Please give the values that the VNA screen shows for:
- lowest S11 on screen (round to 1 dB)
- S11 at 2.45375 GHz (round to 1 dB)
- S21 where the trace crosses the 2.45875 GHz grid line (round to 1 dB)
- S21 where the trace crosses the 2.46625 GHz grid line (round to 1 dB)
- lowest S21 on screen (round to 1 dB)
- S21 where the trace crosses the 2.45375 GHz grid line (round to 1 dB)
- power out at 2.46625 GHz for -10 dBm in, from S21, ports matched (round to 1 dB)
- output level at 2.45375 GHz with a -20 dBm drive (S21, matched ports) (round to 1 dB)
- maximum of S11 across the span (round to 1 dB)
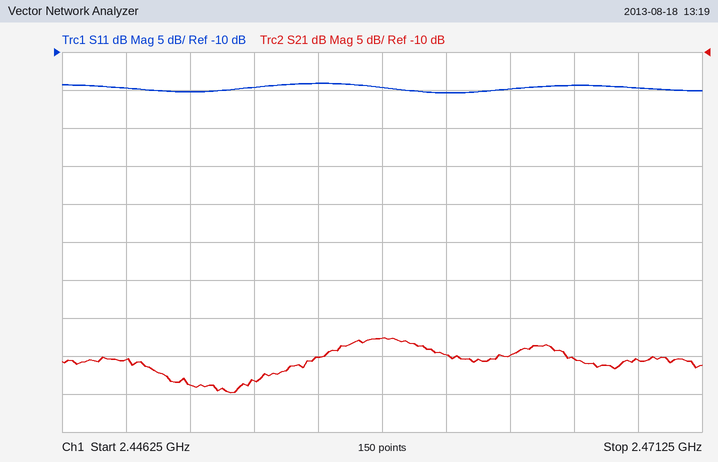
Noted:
-15 dB
-15 dB
-48 dB
-50 dB
-55 dB
-53 dB
-60 dBm
-73 dBm
-14 dB
